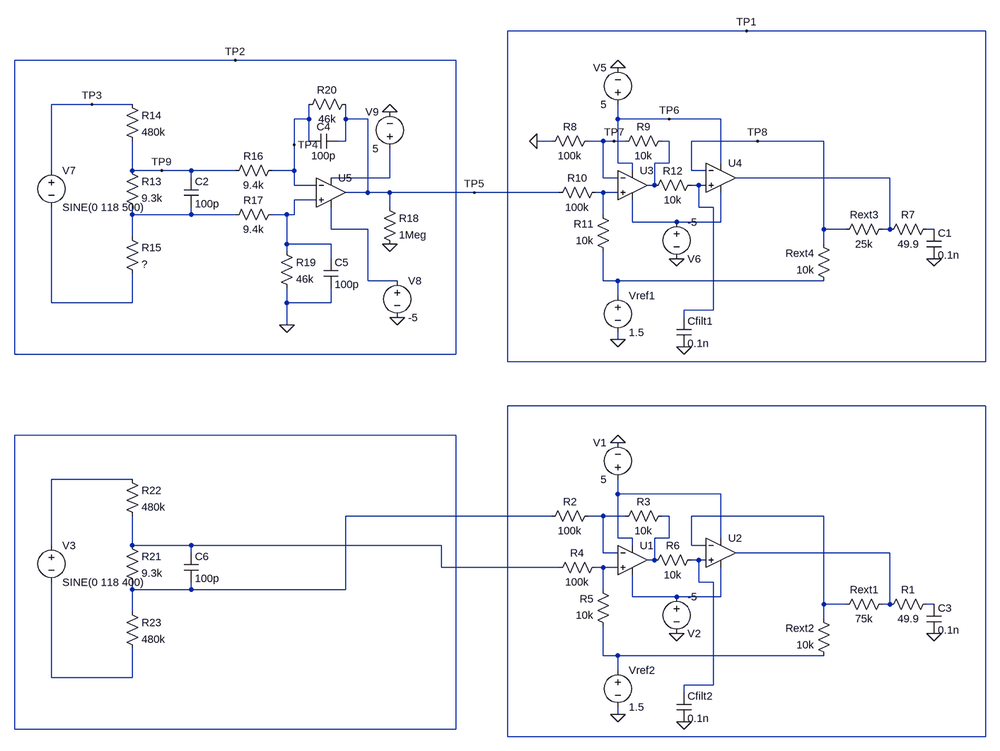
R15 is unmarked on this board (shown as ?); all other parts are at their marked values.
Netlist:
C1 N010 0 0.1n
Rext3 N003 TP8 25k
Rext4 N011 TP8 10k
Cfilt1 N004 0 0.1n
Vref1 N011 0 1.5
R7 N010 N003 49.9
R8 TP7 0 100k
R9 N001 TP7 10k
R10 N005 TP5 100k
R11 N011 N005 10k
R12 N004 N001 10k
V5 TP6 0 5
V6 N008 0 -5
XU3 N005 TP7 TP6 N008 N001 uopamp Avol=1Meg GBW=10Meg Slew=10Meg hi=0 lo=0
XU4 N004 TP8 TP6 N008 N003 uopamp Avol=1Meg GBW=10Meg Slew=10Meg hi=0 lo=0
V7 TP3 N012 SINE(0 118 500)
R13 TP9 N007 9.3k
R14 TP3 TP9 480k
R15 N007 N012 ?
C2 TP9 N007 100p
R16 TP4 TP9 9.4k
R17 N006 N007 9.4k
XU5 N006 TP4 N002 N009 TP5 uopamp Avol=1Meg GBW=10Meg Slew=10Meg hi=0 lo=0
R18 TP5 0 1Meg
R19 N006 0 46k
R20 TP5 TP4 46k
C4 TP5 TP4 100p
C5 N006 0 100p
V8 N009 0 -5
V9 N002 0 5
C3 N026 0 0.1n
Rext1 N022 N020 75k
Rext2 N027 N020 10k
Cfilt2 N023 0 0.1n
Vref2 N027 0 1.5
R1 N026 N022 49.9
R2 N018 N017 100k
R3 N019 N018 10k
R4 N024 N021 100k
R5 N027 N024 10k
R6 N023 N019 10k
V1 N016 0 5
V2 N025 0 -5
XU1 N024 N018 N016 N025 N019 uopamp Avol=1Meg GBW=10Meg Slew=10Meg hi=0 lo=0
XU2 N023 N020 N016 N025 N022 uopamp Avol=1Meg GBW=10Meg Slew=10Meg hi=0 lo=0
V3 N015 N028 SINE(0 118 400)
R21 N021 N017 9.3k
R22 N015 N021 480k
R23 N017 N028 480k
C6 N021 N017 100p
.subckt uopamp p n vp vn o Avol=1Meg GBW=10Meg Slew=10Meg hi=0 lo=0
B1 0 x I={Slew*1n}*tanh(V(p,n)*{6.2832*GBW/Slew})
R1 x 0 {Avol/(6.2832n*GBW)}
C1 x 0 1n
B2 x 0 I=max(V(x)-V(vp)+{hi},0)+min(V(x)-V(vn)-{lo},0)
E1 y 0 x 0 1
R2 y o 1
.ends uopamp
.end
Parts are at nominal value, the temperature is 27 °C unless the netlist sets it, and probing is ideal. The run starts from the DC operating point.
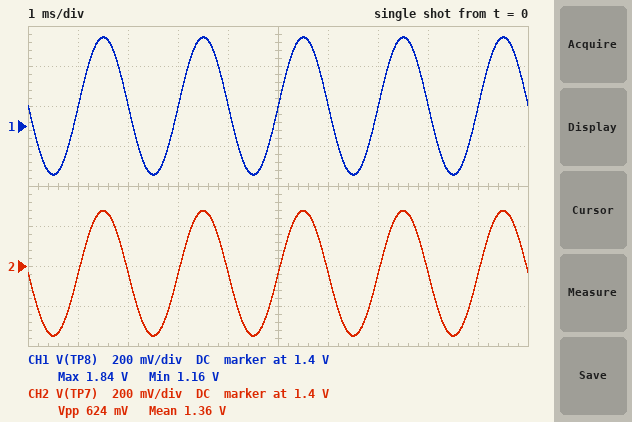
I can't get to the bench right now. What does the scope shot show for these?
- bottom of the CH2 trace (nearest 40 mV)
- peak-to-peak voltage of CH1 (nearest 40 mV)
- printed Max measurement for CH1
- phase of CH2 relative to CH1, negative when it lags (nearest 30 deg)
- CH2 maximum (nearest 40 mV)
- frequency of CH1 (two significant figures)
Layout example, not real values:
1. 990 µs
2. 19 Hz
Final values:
1. 1.04 V
2. 680 mV
3. 1.84 V
4. 0 deg
5. 1.68 V
6. 500 Hz
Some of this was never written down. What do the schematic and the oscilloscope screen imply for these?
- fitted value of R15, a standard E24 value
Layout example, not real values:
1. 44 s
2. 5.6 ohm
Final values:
1. 560 kΩ
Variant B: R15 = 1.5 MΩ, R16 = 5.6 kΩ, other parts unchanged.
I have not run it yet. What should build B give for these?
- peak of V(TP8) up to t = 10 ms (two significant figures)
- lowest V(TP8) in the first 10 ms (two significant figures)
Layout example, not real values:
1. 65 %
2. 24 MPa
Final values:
1. 1.7 V
2. 1.3 V
